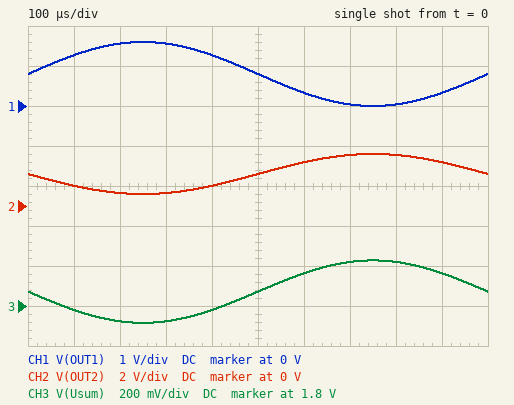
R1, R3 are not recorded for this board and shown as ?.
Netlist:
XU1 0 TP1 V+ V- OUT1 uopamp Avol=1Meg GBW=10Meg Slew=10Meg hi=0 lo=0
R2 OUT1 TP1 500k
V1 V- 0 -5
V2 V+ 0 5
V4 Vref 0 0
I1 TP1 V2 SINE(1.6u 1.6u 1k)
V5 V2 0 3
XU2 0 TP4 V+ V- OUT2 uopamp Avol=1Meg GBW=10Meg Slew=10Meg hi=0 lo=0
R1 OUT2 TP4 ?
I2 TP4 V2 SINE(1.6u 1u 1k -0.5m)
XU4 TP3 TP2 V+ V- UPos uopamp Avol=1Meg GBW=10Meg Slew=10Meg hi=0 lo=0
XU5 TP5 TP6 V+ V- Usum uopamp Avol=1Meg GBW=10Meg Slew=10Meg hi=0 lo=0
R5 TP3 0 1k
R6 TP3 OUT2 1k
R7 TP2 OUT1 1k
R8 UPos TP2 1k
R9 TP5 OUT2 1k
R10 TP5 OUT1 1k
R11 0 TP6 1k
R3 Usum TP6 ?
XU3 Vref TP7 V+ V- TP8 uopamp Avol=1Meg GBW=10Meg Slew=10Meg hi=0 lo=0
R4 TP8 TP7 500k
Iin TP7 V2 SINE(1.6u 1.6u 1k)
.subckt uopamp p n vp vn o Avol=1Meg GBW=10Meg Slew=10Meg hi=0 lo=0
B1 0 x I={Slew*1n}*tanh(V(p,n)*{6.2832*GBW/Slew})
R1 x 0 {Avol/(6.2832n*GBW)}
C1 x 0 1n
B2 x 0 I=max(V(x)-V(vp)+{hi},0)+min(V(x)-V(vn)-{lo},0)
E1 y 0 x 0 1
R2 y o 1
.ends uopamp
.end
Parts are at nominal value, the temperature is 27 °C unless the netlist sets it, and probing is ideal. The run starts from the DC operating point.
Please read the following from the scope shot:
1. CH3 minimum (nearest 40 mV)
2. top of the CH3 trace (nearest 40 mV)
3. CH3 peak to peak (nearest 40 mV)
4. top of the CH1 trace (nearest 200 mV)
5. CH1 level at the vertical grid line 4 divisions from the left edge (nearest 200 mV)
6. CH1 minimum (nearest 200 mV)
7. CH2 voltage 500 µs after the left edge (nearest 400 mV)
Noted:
1.72 V
2.04 V
320 mV
1.6 V
1.2 V
0 V
1.6 V
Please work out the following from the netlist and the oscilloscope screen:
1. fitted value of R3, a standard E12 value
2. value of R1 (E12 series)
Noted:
560 Ω
1 MΩ
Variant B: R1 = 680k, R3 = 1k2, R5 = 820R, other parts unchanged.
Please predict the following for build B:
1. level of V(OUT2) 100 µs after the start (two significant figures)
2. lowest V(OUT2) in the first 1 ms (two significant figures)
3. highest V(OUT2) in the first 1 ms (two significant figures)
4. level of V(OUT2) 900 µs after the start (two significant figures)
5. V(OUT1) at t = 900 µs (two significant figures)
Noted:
690 mV
410 mV
1.8 V
1.5 V
330 mV
